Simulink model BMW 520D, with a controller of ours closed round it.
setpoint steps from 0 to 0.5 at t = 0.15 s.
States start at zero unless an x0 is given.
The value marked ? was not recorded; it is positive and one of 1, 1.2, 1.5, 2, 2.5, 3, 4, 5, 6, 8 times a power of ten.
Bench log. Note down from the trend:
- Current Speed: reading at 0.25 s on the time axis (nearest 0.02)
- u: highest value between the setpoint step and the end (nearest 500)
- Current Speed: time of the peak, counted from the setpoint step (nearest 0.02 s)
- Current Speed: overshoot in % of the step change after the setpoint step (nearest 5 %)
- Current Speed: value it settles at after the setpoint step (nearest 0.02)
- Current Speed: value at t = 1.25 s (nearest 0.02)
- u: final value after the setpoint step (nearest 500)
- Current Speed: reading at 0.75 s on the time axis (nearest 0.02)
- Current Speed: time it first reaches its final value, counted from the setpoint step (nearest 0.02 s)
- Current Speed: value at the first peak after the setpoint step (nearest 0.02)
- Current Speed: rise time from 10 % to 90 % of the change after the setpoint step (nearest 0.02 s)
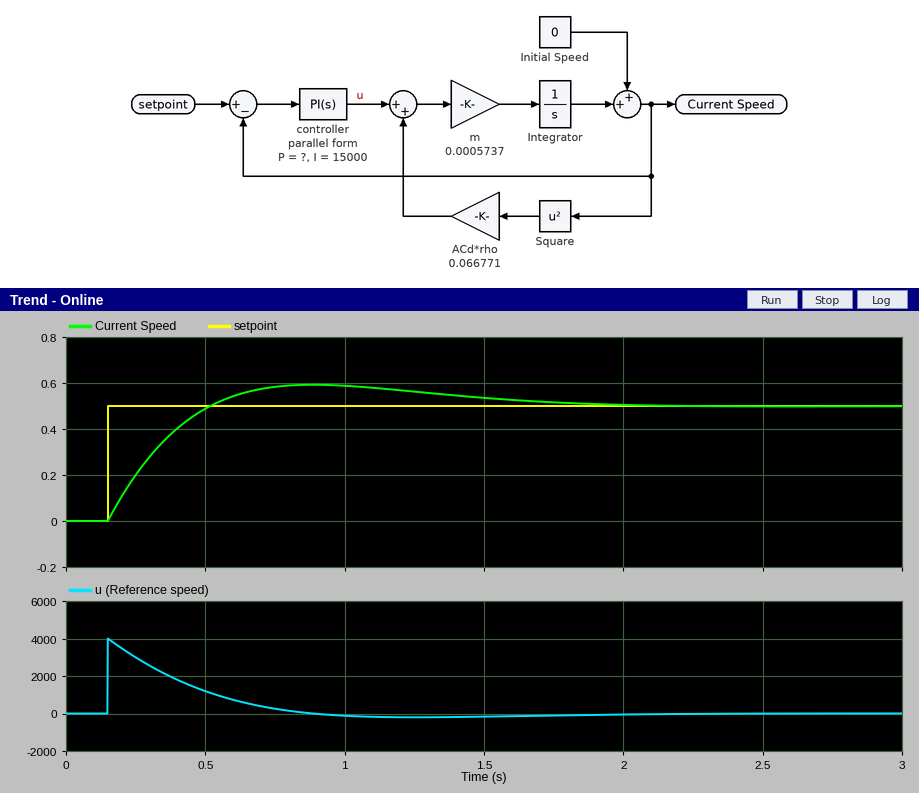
0.20
4000
0.74 s
20 %
0.50
0.56
0
0.58
0.36 s
0.60
0.28 s
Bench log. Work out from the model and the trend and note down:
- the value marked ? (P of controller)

8000
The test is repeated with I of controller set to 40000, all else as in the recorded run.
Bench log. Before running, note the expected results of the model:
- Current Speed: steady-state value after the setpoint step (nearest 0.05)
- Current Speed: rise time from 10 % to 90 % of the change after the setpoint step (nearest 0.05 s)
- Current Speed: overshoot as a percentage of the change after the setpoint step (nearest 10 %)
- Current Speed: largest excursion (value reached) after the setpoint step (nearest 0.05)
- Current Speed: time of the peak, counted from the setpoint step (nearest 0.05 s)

0.50
0.20 s
30 %
0.65
0.50 s
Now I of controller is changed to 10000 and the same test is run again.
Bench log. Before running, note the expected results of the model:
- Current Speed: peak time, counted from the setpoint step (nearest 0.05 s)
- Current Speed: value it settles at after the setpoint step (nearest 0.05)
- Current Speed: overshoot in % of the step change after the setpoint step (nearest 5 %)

0.85 s
0.50
15 %
